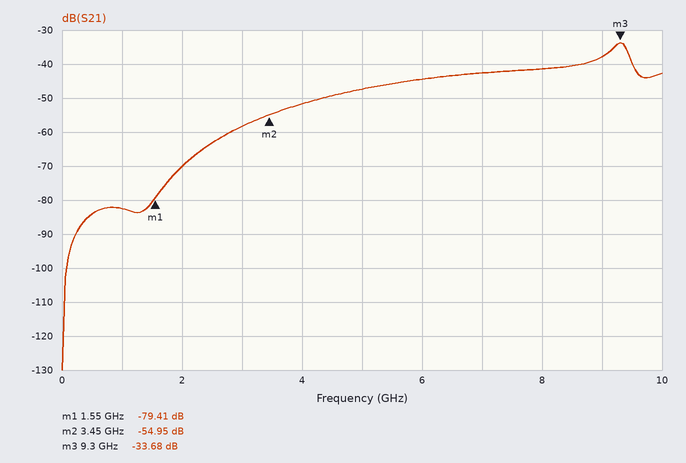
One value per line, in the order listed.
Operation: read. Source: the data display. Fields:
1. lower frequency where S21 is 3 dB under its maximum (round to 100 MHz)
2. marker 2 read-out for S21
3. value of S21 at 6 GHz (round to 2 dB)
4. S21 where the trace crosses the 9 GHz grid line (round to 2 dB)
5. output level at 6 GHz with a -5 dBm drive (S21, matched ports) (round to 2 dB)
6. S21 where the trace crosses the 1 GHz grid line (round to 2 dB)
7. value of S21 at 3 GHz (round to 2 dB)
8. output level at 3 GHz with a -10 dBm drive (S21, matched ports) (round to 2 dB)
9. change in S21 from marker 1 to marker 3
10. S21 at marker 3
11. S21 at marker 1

9.1 GHz
-54.95 dB
-44 dB
-38 dB
-50 dBm
-82 dB
-58 dB
-68 dBm
45.73 dB
-33.68 dB
-79.41 dB
